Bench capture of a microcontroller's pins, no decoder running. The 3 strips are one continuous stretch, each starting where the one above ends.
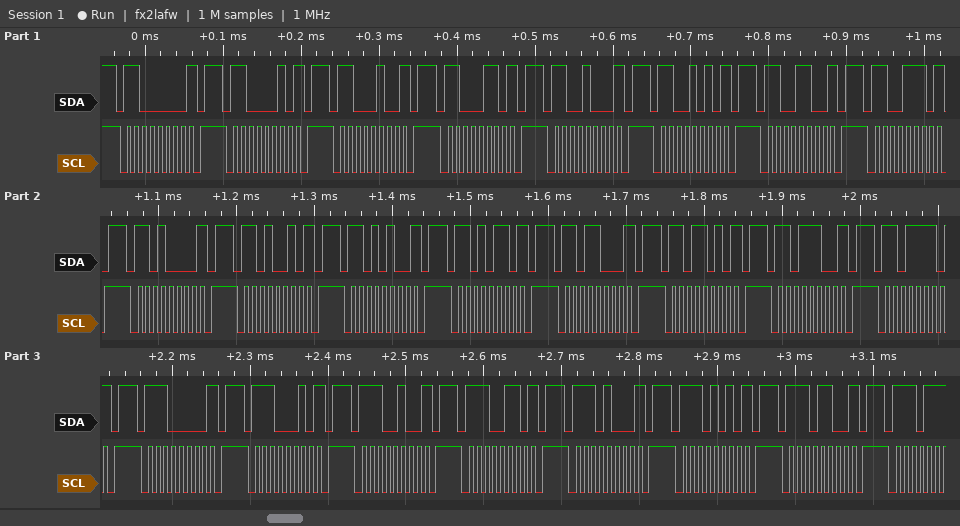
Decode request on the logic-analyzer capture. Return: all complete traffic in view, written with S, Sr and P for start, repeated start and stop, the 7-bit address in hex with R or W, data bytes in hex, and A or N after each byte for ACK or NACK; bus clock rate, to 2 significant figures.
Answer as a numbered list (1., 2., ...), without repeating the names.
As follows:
1. S 60W N P S 61W N P S 62W N P S 63W N P S 64W N P S 65W N P S 66W N P S 67W N P S 68W N P S 69W N P S 6AW N P S 6BW N P S 6CW N P S 6DW N P S 6EW N P S 6FW N P S 70W N P S 71W N P S 72W N P S 73W N P S 74W N P S 75W N P S 76W N P
2. 100 kHz
